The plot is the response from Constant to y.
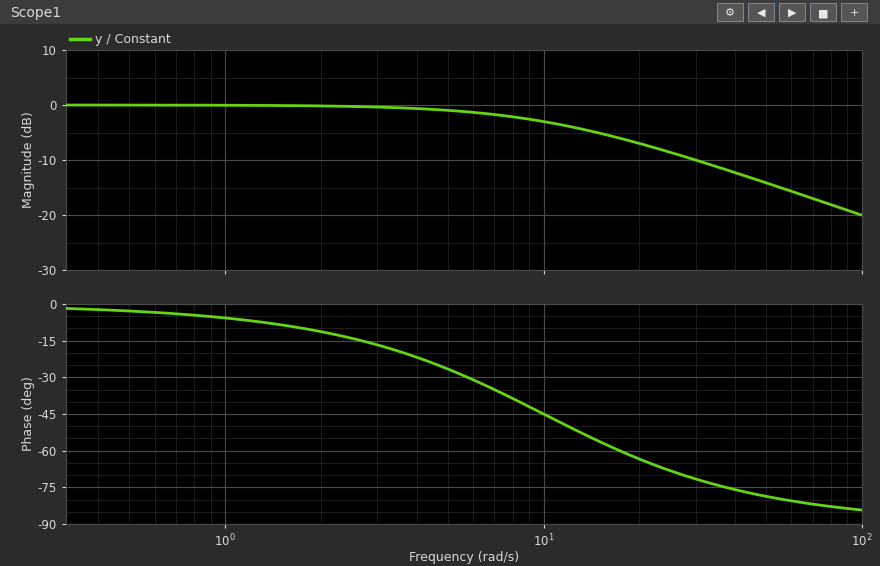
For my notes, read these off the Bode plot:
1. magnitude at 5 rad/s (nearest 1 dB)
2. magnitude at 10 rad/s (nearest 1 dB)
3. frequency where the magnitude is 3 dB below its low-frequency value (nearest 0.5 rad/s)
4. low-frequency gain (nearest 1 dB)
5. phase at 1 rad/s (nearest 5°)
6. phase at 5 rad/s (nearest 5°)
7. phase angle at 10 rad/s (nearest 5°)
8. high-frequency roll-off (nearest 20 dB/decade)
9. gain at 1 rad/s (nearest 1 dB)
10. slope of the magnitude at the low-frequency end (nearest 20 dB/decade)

-1 dB
-3 dB
10.0 rad/s
0 dB
-5°
-25°
-45°
-20 dB/decade
0 dB
0 dB/decade
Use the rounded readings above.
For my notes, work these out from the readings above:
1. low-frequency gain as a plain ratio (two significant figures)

1.0
